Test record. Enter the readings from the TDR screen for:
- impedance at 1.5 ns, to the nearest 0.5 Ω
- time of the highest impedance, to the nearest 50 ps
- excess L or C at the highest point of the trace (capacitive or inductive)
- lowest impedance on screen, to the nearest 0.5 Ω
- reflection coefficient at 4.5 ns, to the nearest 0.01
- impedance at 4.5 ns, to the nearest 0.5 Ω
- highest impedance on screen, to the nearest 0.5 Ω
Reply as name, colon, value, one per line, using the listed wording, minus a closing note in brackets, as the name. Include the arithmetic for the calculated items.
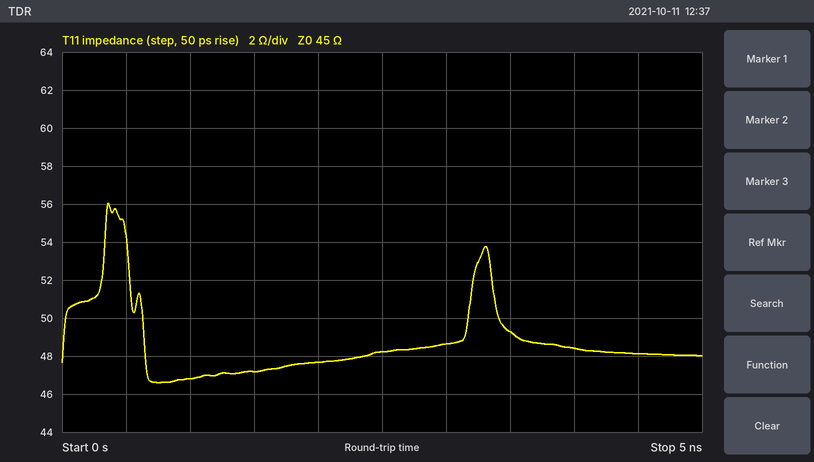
impedance at 1.5 ns, to the nearest 0.5 Ω: 47.0 Ω
time of the highest impedance, to the nearest 50 ps: 350 ps
excess L or C at the highest point of the trace: inductive
lowest impedance on screen, to the nearest 0.5 Ω: 46.5 Ω
reflection coefficient at 4.5 ns, to the nearest 0.01: (48 − 45)/(48 + 45) ≈ +0.03
impedance at 4.5 ns, to the nearest 0.5 Ω: 48.0 Ω
highest impedance on screen, to the nearest 0.5 Ω: 56.0 Ω
